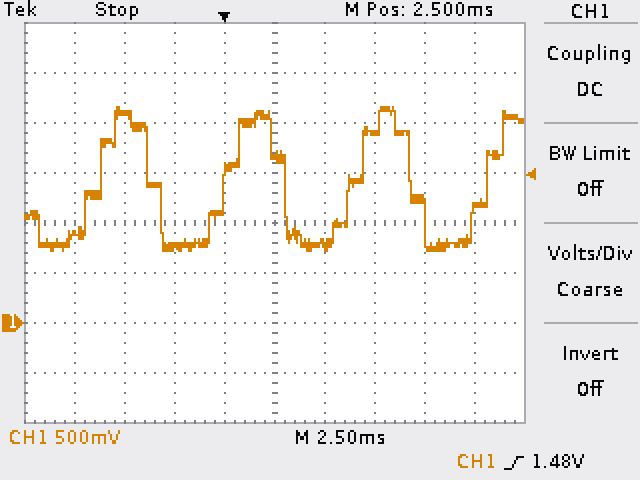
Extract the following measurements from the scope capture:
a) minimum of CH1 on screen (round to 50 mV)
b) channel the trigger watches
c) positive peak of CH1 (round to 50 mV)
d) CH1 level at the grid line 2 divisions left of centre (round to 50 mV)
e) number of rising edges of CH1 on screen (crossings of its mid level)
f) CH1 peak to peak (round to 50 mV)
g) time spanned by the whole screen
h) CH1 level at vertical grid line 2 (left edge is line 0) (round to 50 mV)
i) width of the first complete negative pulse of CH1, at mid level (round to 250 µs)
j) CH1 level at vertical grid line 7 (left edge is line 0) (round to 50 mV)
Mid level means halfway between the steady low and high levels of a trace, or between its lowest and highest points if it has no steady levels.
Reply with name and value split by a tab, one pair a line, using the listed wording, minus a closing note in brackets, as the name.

minimum of CH1 on screen	700 mV
channel the trigger watches	CH1
positive peak of CH1	2.15 V
CH1 level at the grid line 2 divisions left of centre	750 mV
number of rising edges of CH1 on screen	4
CH1 peak to peak	1.45 V
time spanned by the whole screen	25 ms
CH1 level at vertical grid line 2 (left edge is line 0)	2.10 V
width of the first complete negative pulse of CH1, at mid level	3.75 ms
CH1 level at vertical grid line 7 (left edge is line 0)	1.90 V
